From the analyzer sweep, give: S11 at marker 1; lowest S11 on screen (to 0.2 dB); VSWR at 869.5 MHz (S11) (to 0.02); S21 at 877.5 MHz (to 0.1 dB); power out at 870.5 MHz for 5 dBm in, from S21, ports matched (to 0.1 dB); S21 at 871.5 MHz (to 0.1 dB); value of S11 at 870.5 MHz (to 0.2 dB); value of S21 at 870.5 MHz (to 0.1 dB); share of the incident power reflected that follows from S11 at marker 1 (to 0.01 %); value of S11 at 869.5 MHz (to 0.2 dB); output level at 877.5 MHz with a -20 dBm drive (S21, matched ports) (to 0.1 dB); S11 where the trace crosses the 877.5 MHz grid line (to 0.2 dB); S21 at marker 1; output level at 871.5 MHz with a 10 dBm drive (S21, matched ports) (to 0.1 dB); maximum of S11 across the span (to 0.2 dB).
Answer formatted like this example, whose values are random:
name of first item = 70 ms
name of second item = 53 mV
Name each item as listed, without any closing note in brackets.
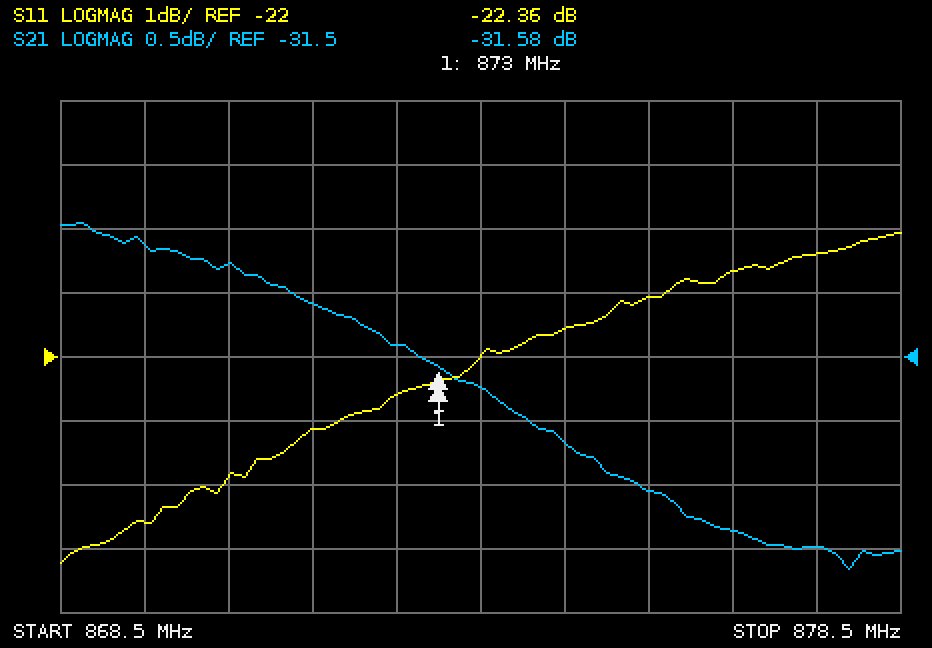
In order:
S11 at marker 1 = -22.36 dB
lowest S11 on screen = -25.2 dB
VSWR at 869.5 MHz (S11) = 1.12
S21 at 877.5 MHz = -33.0 dB
power out at 870.5 MHz for 5 dBm in, from S21, ports matched = -25.8 dBm
S21 at 871.5 MHz = -31.1 dB
value of S11 at 870.5 MHz = -23.8 dB
value of S21 at 870.5 MHz = -30.8 dB
share of the incident power reflected that follows from S11 at marker 1 = 0.58 %
value of S11 at 869.5 MHz = -24.6 dB
output level at 877.5 MHz with a -20 dBm drive (S21, matched ports) = -53.0 dBm
S11 where the trace crosses the 877.5 MHz grid line = -20.4 dB
S21 at marker 1 = -31.58 dB
output level at 871.5 MHz with a 10 dBm drive (S21, matched ports) = -21.1 dBm
maximum of S11 across the span = -20.0 dB
